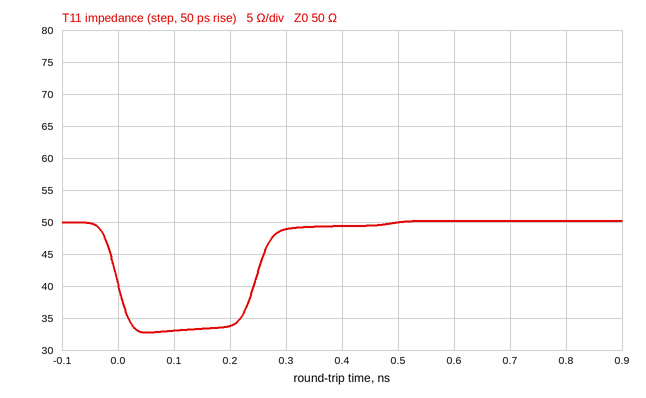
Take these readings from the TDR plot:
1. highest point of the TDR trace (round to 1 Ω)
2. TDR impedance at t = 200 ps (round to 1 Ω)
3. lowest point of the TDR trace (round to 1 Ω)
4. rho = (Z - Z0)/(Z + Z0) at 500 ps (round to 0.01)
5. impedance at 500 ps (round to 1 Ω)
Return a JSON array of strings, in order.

["50 Ω", "34 Ω", "33 Ω", "0.00", "50 Ω"]
